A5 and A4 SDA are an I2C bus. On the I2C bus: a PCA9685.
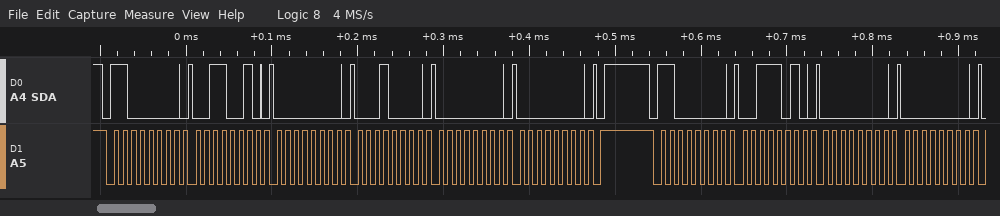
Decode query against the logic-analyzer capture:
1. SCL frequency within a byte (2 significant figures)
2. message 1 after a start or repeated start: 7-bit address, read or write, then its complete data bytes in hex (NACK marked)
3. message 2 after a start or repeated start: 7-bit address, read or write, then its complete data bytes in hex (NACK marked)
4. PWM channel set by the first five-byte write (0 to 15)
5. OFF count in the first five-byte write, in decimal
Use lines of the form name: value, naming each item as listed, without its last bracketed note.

SCL frequency within a byte: 100 kHz
message 1 after a start or repeated start: 7-bit address, read or write, then its complete data bytes in hex: 0x60 write: 32 00 10 00 00
message 2 after a start or repeated start: 7-bit address, read or write, then its complete data bytes in hex: 0x60 write: 3A 00 00
PWM channel set by the first five-byte write: 11
OFF count in the first five-byte write, in decimal: 0
